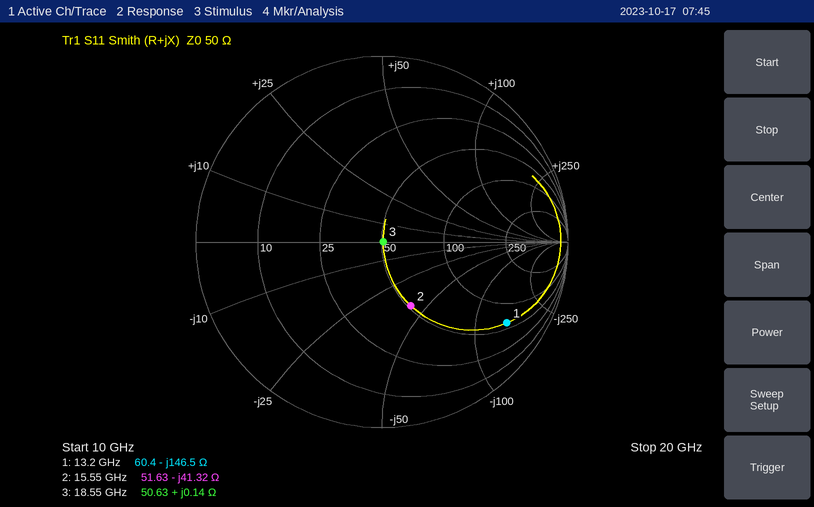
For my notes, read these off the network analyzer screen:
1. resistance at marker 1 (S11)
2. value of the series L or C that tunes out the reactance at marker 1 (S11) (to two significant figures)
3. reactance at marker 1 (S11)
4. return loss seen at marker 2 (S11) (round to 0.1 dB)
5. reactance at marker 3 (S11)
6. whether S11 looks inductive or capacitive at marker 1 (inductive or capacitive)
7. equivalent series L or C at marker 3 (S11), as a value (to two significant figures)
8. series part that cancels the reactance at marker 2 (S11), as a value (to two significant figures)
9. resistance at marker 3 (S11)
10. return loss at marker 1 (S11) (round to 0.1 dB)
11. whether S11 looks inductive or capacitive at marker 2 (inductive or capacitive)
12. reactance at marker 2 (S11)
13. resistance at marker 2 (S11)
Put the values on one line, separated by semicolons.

60.4 Ω; 1.8 nH; -146.5 Ω; 8.5 dB; +0.14 Ω; capacitive; 1.2 pH; 420 pH; 50.63 Ω; 1.9 dB; capacitive; -41.32 Ω; 51.63 Ω
